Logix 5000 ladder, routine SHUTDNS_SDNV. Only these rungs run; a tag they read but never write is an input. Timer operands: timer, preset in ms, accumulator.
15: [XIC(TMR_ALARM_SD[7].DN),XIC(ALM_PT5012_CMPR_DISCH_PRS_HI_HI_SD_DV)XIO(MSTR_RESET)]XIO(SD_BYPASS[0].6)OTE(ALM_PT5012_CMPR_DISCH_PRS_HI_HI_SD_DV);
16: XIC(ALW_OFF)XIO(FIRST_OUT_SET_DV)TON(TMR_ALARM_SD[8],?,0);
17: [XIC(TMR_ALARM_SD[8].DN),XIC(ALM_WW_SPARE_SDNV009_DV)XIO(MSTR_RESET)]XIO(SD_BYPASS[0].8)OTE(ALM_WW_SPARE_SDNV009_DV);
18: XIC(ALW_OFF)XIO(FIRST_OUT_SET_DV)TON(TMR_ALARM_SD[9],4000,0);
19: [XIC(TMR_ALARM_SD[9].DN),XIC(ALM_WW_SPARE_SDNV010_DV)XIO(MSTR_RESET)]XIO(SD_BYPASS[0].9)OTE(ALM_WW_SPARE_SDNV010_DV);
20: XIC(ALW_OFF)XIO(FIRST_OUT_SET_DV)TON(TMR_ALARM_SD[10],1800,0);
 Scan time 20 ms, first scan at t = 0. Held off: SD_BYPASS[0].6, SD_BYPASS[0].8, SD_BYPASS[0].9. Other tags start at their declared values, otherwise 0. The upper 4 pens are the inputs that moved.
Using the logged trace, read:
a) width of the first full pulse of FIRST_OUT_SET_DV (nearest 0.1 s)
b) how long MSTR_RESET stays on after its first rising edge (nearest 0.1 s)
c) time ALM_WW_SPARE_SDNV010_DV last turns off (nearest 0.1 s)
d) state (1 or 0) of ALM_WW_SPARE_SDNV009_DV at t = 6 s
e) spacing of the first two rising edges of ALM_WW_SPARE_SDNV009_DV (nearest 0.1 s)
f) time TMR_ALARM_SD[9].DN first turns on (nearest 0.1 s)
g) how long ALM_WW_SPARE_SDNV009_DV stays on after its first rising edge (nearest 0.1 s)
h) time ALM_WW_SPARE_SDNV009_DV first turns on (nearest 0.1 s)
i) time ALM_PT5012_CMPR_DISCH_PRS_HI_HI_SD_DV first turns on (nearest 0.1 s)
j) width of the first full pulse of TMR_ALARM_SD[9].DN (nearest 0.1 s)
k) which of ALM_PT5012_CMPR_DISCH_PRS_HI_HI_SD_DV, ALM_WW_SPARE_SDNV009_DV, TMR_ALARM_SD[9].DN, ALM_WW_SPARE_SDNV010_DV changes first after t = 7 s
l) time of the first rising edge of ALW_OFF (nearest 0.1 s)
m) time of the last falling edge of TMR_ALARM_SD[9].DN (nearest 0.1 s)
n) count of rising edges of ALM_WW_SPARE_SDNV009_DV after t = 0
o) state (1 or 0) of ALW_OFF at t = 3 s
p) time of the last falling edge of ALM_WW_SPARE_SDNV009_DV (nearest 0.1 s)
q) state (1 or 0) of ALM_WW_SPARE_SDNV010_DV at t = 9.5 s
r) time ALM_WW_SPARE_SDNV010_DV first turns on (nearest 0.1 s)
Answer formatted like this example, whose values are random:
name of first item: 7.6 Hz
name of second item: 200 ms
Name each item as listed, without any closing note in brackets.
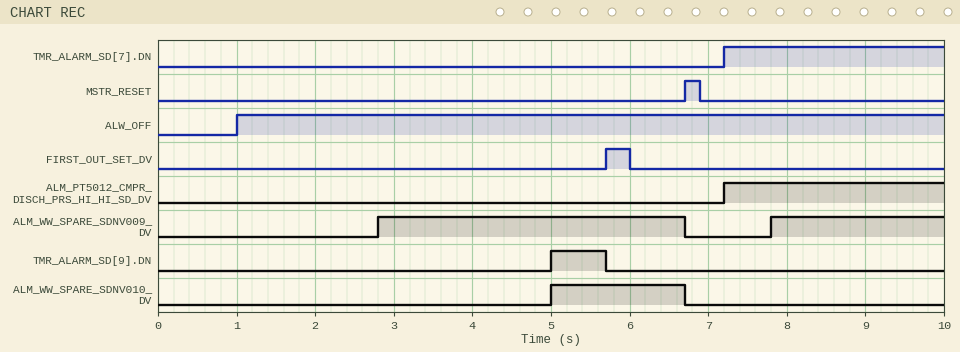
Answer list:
width of the first full pulse of FIRST_OUT_SET_DV: 0.3 s
how long MSTR_RESET stays on after its first rising edge: 0.2 s
time ALM_WW_SPARE_SDNV010_DV last turns off: 6.7 s
state (1 or 0) of ALM_WW_SPARE_SDNV009_DV at t = 6 s: 1
spacing of the first two rising edges of ALM_WW_SPARE_SDNV009_DV: 5.0 s
time TMR_ALARM_SD[9].DN first turns on: 5.0 s
how long ALM_WW_SPARE_SDNV009_DV stays on after its first rising edge: 3.9 s
time ALM_WW_SPARE_SDNV009_DV first turns on: 2.8 s
time ALM_PT5012_CMPR_DISCH_PRS_HI_HI_SD_DV first turns on: 7.2 s
width of the first full pulse of TMR_ALARM_SD[9].DN: 0.7 s
which of ALM_PT5012_CMPR_DISCH_PRS_HI_HI_SD_DV, ALM_WW_SPARE_SDNV009_DV, TMR_ALARM_SD[9].DN, ALM_WW_SPARE_SDNV010_DV changes first after t = 7 s: ALM_PT5012_CMPR_DISCH_PRS_HI_HI_SD_DV
time of the first rising edge of ALW_OFF: 1.0 s
time of the last falling edge of TMR_ALARM_SD[9].DN: 5.7 s
count of rising edges of ALM_WW_SPARE_SDNV009_DV after t = 0: 2
state (1 or 0) of ALW_OFF at t = 3 s: 1
time of the last falling edge of ALM_WW_SPARE_SDNV009_DV: 6.7 s
state (1 or 0) of ALM_WW_SPARE_SDNV010_DV at t = 9.5 s: 0
time ALM_WW_SPARE_SDNV010_DV first turns on: 5.0 s
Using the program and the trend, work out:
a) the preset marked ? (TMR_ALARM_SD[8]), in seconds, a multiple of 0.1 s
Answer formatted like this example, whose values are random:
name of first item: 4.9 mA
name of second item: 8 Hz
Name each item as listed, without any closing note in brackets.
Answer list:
the preset marked ? (TMR_ALARM_SD[8]), in seconds, a multiple of 0.1 s: 1.8 s
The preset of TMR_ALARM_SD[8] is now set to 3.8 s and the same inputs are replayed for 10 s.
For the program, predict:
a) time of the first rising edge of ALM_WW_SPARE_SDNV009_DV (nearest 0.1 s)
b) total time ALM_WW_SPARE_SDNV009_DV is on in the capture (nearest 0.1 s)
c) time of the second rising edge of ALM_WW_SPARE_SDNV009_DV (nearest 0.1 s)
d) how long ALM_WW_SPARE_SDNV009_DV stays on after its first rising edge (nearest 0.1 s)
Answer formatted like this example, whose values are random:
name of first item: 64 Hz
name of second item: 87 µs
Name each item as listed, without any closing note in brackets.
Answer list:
time of the first rising edge of ALM_WW_SPARE_SDNV009_DV: 4.8 s
total time ALM_WW_SPARE_SDNV009_DV is on in the capture: 2.1 s
time of the second rising edge of ALM_WW_SPARE_SDNV009_DV: 9.8 s
how long ALM_WW_SPARE_SDNV009_DV stays on after its first rising edge: 1.9 s
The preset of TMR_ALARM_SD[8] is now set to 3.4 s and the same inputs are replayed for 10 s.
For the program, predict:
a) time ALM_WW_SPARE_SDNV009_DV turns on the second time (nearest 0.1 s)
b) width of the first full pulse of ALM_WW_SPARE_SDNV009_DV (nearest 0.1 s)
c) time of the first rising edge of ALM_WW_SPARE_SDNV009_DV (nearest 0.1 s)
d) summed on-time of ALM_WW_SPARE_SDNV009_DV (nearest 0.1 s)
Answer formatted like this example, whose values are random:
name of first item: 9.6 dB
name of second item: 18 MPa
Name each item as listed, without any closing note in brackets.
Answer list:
time ALM_WW_SPARE_SDNV009_DV turns on the second time: 9.4 s
width of the first full pulse of ALM_WW_SPARE_SDNV009_DV: 2.3 s
time of the first rising edge of ALM_WW_SPARE_SDNV009_DV: 4.4 s
summed on-time of ALM_WW_SPARE_SDNV009_DV: 2.9 s
